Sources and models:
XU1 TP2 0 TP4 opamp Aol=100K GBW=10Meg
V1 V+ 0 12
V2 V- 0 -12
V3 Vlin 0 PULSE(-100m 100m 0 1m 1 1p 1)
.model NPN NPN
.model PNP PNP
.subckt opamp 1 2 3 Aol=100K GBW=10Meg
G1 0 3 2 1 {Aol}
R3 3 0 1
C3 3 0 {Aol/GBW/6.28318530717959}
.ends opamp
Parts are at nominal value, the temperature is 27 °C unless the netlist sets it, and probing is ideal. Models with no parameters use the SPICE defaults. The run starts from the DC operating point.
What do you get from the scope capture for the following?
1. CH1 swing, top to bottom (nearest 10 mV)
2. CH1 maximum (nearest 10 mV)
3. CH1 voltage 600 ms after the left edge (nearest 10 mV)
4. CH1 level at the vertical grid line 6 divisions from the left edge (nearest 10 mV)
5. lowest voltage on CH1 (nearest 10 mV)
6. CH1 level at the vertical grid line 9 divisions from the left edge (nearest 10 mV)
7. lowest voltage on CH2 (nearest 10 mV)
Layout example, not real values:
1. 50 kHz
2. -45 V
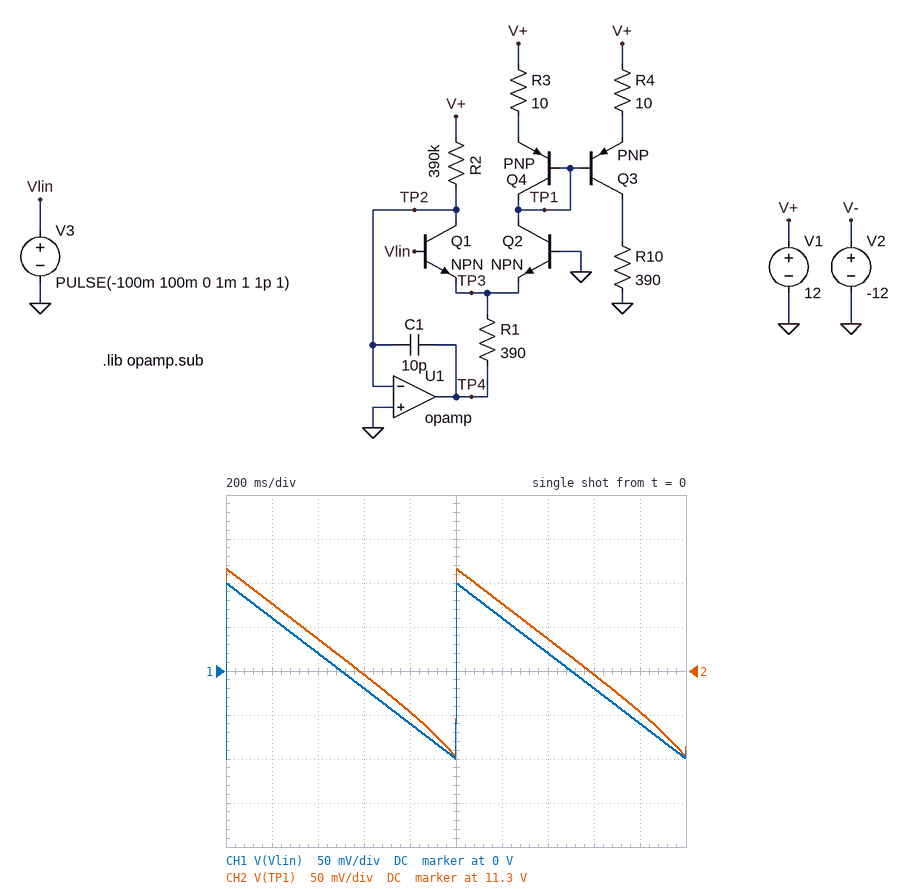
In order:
1. 200 mV
2. 100 mV
3. -20 mV
4. 60 mV
5. -100 mV
6. -60 mV
7. 11.20 V
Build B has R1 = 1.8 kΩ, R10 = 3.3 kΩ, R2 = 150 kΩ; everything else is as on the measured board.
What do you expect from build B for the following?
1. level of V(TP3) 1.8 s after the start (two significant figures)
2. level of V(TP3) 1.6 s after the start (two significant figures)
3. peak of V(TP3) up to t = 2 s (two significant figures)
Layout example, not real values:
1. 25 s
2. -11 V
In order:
1. -770 mV
2. -730 mV
3. -610 mV
